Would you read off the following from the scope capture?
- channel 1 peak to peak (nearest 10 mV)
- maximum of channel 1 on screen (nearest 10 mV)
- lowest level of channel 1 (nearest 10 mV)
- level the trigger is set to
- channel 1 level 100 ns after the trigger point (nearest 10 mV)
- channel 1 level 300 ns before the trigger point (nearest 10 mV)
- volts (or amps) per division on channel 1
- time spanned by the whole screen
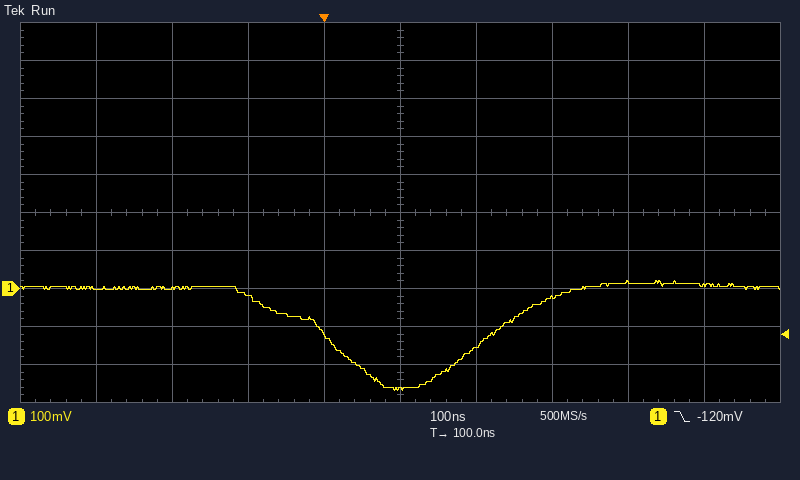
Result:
290 mV
20 mV
-270 mV
-120 mV
-260 mV
0 mV
100 mV
1 µs
